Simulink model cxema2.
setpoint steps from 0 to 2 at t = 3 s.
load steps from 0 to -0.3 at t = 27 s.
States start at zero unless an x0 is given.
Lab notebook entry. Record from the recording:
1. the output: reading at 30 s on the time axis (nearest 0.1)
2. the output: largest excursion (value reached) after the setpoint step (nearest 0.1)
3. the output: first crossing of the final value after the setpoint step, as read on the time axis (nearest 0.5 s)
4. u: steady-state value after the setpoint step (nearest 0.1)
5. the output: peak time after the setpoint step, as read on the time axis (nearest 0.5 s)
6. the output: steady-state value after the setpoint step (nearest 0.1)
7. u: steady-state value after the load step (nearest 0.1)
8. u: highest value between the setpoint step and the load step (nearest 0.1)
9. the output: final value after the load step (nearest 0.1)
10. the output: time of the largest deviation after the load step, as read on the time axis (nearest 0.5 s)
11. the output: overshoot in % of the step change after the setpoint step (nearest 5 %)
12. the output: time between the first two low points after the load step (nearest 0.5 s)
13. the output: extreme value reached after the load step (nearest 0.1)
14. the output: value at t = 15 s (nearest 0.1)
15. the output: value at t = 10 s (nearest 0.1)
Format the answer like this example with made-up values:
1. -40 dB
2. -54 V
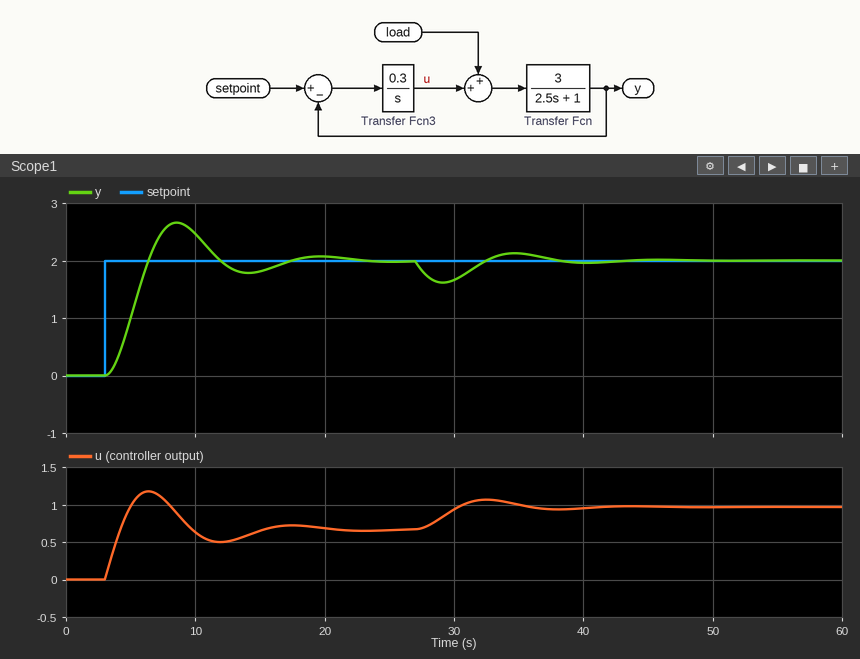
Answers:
1. 1.7
2. 2.7
3. 6.5 s
4. 0.7
5. 8.5 s
6. 2.0
7. 1.0
8. 1.2
9. 2.0
10. 29.0 s
11. 35 %
12. 11.0 s
13. 1.6
14. 1.8
15. 2.5
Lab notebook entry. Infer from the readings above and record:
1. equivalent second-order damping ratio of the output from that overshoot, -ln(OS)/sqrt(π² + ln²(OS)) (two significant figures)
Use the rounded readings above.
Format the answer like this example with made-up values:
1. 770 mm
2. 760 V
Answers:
1. 0.32
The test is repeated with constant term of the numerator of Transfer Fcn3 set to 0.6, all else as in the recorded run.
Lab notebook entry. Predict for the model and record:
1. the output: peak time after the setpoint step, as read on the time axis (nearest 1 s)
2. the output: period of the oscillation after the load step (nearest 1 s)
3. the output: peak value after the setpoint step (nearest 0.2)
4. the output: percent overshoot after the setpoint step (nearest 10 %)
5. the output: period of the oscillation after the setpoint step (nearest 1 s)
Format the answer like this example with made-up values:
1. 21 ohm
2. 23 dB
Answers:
1. 7 s
2. 8 s
3. 3.0
4. 50 %
5. 8 s
